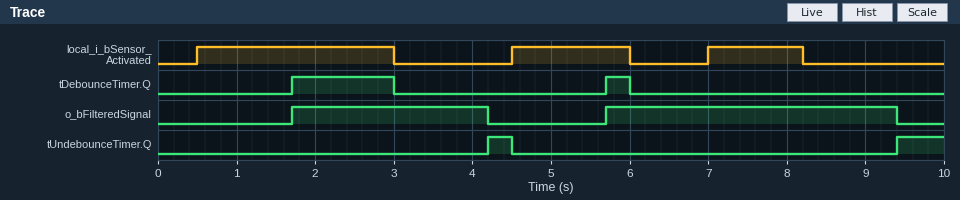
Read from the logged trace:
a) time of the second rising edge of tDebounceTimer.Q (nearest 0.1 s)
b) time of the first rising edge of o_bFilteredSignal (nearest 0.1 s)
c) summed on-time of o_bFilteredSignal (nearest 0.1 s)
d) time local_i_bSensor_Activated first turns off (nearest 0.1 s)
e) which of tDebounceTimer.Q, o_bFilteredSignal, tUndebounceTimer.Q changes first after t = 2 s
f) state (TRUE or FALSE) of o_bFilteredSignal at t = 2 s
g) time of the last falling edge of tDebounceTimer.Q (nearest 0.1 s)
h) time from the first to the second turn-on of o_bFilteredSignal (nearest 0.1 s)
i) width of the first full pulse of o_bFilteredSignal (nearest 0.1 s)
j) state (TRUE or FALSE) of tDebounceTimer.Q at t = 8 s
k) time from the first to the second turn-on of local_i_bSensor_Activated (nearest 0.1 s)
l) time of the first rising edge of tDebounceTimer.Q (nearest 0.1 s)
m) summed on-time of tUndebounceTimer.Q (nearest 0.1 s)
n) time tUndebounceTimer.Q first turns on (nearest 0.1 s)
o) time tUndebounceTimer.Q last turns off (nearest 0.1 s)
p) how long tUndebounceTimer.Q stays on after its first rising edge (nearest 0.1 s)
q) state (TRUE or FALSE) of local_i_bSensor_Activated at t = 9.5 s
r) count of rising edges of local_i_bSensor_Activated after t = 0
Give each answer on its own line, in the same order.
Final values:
5.7 s
1.7 s
6.2 s
3.0 s
tDebounceTimer.Q
TRUE
6.0 s
4.0 s
2.5 s
FALSE
4.0 s
1.7 s
0.9 s
4.2 s
4.5 s
0.3 s
FALSE
3
